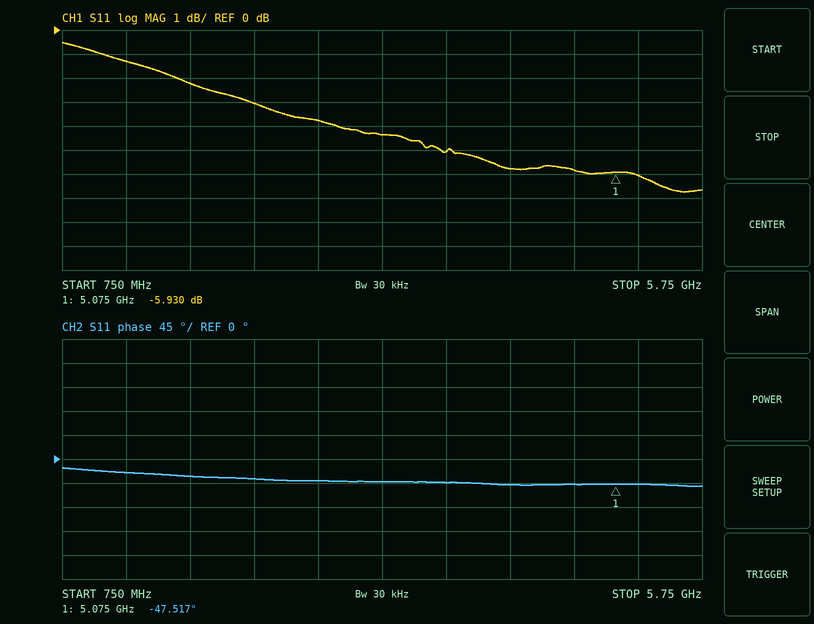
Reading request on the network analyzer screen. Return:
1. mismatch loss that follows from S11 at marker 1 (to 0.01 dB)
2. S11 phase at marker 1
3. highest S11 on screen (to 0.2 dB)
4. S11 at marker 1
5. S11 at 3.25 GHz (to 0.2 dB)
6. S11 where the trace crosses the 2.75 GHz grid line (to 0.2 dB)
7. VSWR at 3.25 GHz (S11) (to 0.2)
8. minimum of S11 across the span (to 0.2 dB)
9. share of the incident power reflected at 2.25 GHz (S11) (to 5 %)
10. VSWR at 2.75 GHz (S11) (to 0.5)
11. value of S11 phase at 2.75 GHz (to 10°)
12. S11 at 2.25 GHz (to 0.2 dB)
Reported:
1.28 dB
-47.517°
-0.6 dB
-5.930 dB
-4.4 dB
-3.8 dB
4.0
-6.8 dB
50 %
4.5
-40°
-3.0 dB
